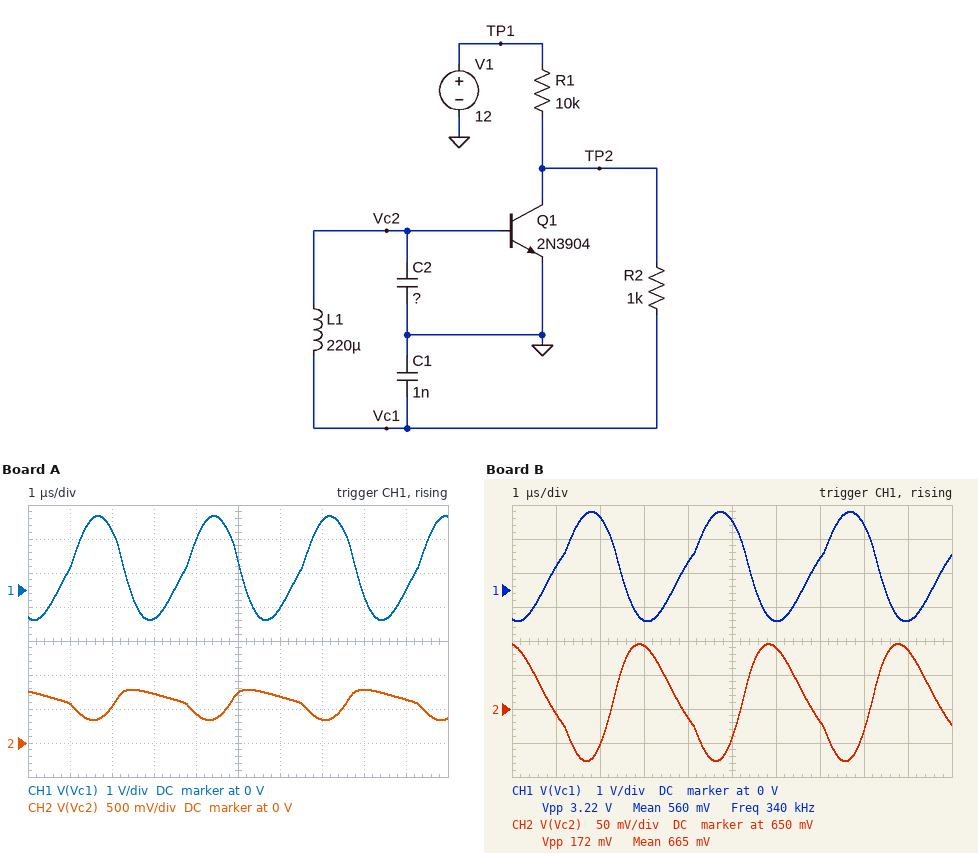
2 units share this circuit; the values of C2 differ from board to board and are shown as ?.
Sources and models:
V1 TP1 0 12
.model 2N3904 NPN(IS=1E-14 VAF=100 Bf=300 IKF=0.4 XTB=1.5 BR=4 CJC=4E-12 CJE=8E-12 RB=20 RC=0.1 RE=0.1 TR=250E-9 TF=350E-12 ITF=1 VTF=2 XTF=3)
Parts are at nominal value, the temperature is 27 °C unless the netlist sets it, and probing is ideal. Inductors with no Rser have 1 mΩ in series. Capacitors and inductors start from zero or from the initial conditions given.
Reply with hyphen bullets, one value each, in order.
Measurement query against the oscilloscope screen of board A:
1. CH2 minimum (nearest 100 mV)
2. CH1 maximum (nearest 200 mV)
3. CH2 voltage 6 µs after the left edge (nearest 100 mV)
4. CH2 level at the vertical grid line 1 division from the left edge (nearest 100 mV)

- 300 mV
- 2.2 V
- 700 mV
- 600 mV
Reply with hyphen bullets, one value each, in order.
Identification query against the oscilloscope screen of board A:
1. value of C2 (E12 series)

- 3.9 nF
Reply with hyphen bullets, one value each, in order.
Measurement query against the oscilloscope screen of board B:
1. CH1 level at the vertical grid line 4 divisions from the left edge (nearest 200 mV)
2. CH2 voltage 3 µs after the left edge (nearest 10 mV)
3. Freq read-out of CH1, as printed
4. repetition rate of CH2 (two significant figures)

- 800 mV
- 740 mV
- 340 kHz
- 340 kHz
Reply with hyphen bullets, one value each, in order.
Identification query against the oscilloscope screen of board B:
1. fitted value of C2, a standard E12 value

- 15 nF
